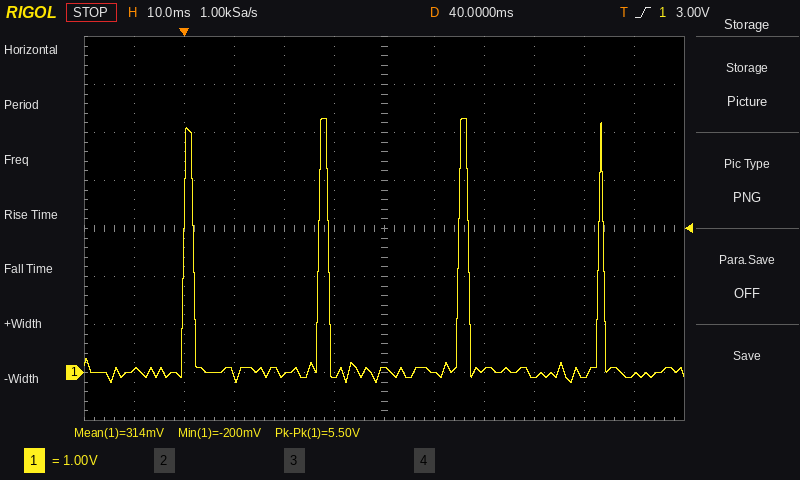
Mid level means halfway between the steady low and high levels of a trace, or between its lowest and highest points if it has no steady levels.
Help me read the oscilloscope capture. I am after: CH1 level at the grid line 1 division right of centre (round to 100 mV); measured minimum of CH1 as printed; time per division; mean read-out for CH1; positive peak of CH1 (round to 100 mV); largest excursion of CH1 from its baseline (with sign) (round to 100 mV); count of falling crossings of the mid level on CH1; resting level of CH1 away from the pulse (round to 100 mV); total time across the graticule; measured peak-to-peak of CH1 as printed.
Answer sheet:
0.0 V
-200 mV
10 ms
314 mV
5.3 V
+5.3 V
4
0.0 V
120 ms
5.50 V
